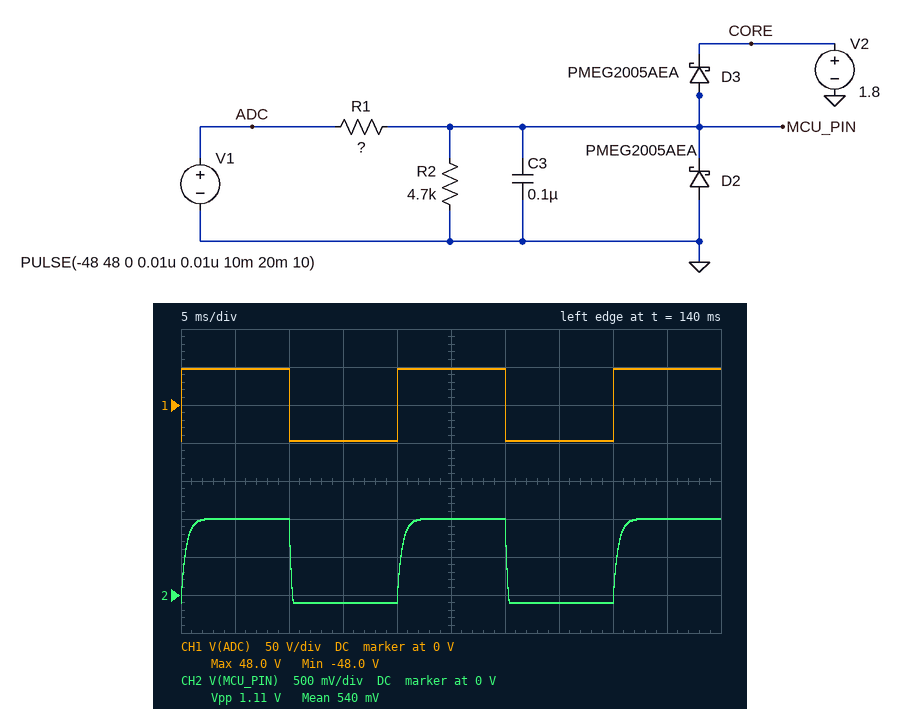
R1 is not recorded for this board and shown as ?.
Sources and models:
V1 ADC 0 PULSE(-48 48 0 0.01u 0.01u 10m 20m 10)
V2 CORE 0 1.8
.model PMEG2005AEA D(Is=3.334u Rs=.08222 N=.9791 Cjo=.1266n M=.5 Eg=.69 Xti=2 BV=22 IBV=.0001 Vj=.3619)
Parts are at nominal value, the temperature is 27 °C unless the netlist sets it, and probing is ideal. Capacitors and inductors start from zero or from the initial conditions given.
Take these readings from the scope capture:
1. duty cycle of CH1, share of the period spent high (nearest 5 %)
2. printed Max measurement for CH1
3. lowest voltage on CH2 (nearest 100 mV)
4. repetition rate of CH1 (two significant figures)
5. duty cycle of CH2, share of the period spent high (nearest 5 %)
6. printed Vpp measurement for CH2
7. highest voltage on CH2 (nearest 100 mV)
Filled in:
50 %
48.0 V
-100 mV
50 Hz
50 %
1.11 V
1.0 V
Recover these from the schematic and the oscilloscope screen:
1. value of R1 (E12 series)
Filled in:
220 kΩ
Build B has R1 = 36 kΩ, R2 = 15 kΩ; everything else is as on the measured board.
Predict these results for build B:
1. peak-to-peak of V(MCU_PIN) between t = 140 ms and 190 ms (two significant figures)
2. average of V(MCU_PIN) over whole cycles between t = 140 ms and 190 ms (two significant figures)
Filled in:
2.1 V
900 mV
